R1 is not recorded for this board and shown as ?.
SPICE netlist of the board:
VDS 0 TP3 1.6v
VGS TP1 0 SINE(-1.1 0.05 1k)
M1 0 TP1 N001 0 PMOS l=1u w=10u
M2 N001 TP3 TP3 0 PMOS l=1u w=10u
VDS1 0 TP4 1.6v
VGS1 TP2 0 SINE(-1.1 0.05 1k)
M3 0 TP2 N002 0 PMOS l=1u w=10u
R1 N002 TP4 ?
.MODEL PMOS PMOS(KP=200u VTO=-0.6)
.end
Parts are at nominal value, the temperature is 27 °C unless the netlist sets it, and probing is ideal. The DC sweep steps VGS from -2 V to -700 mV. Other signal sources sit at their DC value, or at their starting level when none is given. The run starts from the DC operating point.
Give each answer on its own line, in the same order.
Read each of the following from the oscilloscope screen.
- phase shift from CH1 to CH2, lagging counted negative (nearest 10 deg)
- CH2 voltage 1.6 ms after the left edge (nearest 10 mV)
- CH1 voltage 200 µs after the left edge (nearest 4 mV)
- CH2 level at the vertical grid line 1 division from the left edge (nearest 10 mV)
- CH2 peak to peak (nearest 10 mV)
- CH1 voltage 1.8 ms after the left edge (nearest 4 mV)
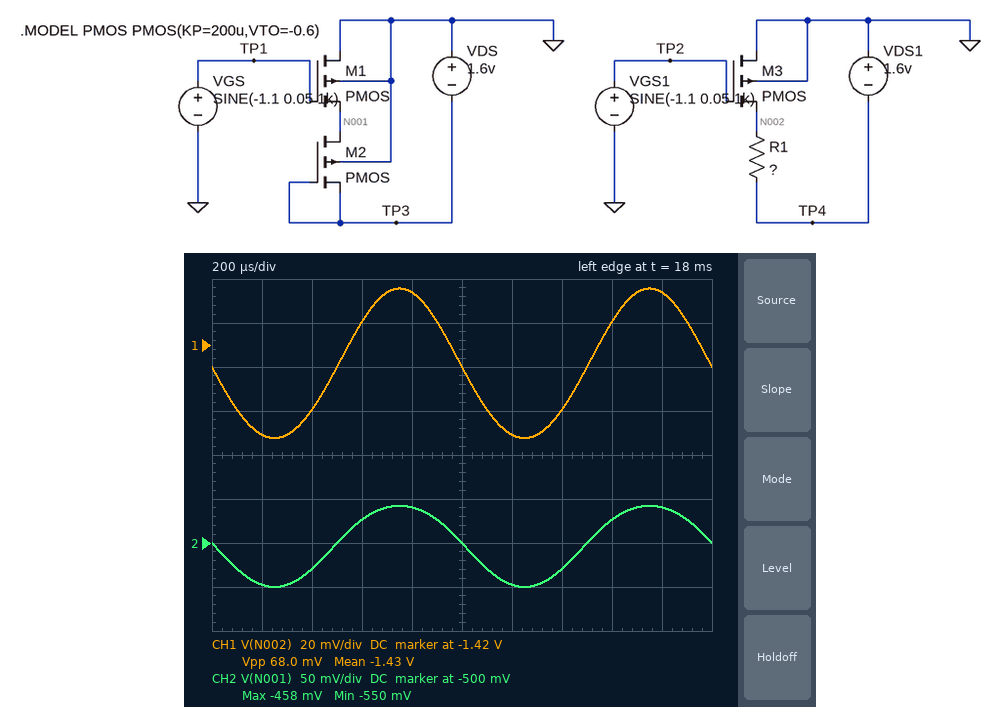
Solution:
0 deg
-470 mV
-1.460 V
-550 mV
90 mV
-1.396 V
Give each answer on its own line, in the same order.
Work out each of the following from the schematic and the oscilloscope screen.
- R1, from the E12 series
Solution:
680 Ω
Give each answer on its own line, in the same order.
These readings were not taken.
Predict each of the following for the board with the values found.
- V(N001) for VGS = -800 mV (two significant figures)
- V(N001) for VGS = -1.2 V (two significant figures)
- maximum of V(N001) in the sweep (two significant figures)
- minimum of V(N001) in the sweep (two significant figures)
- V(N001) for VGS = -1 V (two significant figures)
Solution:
-800 mV
-430 mV
-230 mV
-900 mV
-600 mV
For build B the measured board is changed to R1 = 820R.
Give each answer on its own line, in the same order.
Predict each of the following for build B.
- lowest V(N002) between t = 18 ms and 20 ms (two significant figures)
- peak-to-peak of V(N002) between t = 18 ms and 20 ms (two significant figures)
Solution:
-1.4 V
82 mV
